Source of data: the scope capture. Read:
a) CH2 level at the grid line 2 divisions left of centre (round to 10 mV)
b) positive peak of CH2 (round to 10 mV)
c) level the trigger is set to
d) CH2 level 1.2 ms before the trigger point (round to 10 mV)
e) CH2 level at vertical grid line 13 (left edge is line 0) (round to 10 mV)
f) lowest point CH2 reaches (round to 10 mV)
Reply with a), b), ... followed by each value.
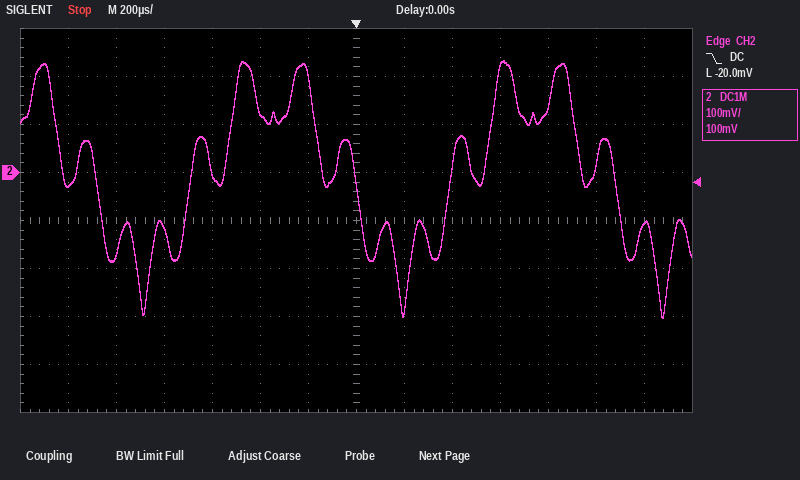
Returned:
a) 130 mV
b) 230 mV
c) -20.0 mV
d) -30 mV
e) -110 mV
f) -300 mV
